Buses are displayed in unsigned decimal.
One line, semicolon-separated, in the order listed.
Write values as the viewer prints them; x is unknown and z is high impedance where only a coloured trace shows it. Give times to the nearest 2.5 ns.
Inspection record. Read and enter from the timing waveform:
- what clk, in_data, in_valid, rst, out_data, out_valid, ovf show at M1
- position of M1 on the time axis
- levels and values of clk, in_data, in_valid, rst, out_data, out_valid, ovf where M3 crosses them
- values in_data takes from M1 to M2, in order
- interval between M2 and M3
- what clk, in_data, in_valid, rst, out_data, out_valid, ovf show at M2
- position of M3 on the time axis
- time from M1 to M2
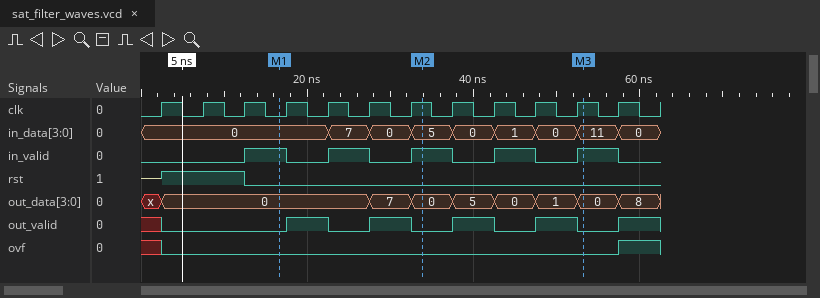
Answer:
clk=0, in_data=0, in_valid=1, rst=0, out_data=0, out_valid=0, ovf=0; 17.5 ns; clk=1, in_data=11, in_valid=1, rst=0, out_data=0, out_valid=0, ovf=0; 0, 7, 0, 5; 20 ns; clk=1, in_data=5, in_valid=1, rst=0, out_data=0, out_valid=0, ovf=0; 52.5 ns; 17.5 ns
